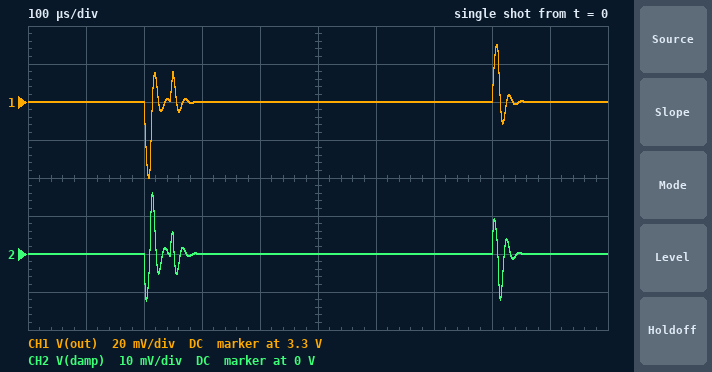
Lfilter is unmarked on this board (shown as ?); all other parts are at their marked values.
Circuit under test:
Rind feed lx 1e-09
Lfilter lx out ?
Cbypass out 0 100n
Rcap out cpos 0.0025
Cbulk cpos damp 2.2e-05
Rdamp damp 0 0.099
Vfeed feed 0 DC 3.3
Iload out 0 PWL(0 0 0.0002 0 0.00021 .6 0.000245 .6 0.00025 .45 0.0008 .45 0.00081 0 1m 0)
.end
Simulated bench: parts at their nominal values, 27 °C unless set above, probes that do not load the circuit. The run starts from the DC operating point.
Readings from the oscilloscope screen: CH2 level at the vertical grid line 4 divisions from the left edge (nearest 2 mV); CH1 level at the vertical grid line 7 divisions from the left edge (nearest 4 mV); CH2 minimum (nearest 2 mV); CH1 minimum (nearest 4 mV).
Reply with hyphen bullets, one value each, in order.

- 0 V
- 3.300 V
- -12 mV
- 3.260 V
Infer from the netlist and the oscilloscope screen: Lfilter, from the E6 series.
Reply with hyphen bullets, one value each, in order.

- 470 nH
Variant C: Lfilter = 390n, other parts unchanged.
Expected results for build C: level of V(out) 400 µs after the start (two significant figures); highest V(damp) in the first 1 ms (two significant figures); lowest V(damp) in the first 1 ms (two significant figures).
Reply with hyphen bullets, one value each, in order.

- 3.3 V
- 14 mV
- -11 mV
